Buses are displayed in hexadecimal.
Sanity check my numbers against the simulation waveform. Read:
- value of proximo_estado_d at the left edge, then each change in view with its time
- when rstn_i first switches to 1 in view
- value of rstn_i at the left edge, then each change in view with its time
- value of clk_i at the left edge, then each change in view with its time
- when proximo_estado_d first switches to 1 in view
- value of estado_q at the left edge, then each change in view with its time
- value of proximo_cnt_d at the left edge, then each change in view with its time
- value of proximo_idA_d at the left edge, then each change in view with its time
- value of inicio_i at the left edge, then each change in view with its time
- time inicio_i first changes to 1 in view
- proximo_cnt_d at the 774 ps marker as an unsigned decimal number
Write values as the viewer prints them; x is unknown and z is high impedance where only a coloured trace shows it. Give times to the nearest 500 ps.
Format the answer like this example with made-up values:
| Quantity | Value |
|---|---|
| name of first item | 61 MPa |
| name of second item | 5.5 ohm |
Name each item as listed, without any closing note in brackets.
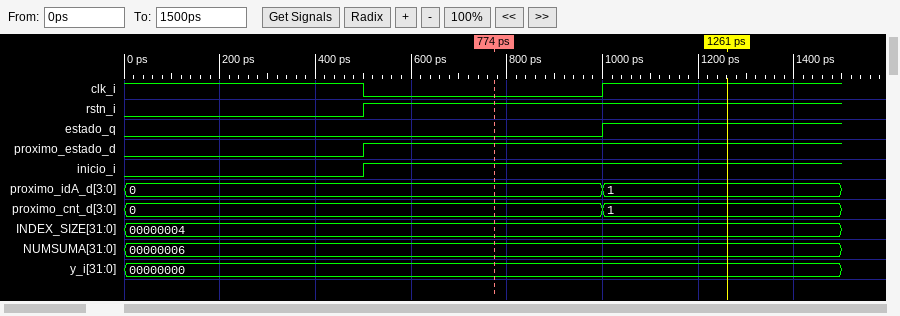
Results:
| Quantity | Value |
|---|---|
| value of proximo_estado_d at the left edge, then each change in view with its time | 0, 1 at 500 ps |
| when rstn_i first switches to 1 in view | 500 ps |
| value of rstn_i at the left edge, then each change in view with its time | 0, 1 at 500 ps |
| value of clk_i at the left edge, then each change in view with its time | 1, 0 at 500 ps, 1 at 1000 ps |
| when proximo_estado_d first switches to 1 in view | 500 ps |
| value of estado_q at the left edge, then each change in view with its time | 0, 1 at 1000 ps |
| value of proximo_cnt_d at the left edge, then each change in view with its time | 0, 1 at 1000 ps |
| value of proximo_idA_d at the left edge, then each change in view with its time | 0, 1 at 1000 ps |
| value of inicio_i at the left edge, then each change in view with its time | 0, 1 at 500 ps |
| time inicio_i first changes to 1 in view | 500 ps |
| proximo_cnt_d at the 774 ps marker as an unsigned decimal number | 0 |
